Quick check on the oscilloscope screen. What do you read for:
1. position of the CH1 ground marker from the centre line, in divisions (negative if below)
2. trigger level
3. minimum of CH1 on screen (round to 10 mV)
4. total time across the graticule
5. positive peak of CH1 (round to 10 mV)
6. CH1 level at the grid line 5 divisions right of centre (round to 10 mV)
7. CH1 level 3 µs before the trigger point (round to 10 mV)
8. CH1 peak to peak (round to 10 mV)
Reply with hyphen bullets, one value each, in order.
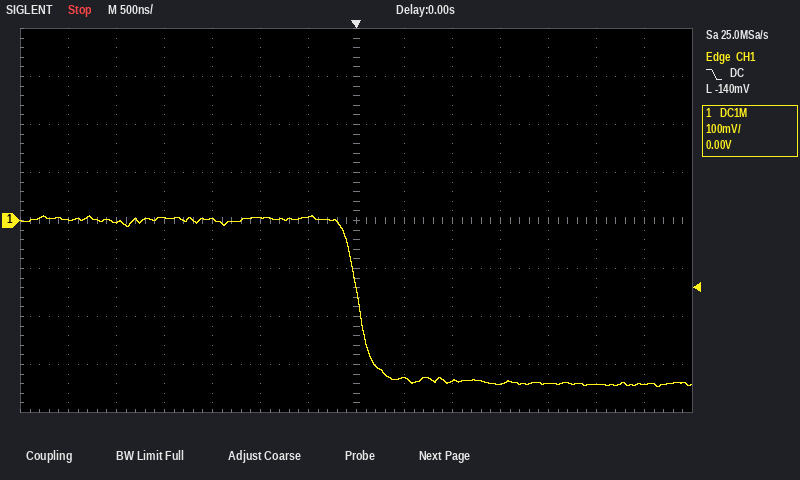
- 0.0 div
- -140 mV
- -350 mV
- 7 µs
- 10 mV
- -340 mV
- 0 mV
- 360 mV
